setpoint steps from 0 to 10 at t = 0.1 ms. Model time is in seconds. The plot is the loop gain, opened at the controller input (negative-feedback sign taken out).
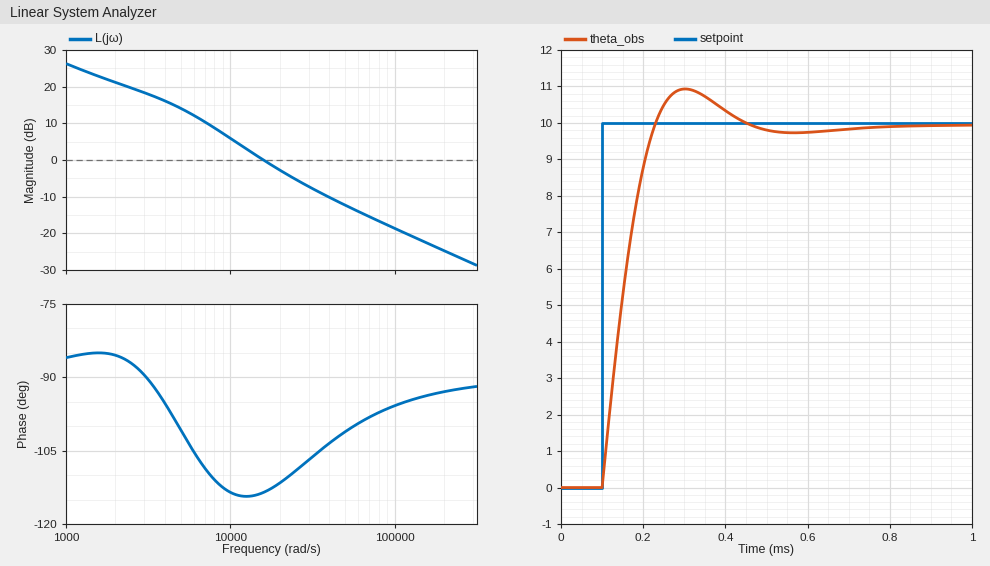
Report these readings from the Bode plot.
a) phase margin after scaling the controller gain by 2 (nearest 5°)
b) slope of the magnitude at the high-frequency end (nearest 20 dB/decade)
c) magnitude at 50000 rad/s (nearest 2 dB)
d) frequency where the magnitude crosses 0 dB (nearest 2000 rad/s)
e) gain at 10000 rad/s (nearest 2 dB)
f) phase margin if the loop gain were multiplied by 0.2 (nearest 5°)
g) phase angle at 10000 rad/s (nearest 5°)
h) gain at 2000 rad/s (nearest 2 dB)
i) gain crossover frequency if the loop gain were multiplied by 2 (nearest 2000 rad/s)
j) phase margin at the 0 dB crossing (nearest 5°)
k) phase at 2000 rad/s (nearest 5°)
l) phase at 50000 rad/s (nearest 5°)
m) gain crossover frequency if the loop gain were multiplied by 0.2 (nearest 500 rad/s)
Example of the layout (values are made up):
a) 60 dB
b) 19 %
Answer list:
a) 70°
b) -20 dB/decade
c) -12 dB
d) 16000 rad/s
e) 6 dB
f) 80°
g) -115°
h) 22 dB
i) 26000 rad/s
j) 65°
k) -85°
l) -100°
m) 5000 rad/s
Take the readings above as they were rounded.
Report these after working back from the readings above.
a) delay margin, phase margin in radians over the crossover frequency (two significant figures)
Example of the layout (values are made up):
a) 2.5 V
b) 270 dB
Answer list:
a) 0.000071 s
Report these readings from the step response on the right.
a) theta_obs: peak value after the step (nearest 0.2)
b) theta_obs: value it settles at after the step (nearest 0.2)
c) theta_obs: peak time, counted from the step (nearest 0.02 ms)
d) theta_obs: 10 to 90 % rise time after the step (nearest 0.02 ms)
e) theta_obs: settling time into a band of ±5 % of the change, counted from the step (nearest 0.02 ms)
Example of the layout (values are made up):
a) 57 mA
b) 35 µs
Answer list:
a) 11.0
b) 10.0
c) 0.20 ms
d) 0.10 ms
e) 0.28 ms
